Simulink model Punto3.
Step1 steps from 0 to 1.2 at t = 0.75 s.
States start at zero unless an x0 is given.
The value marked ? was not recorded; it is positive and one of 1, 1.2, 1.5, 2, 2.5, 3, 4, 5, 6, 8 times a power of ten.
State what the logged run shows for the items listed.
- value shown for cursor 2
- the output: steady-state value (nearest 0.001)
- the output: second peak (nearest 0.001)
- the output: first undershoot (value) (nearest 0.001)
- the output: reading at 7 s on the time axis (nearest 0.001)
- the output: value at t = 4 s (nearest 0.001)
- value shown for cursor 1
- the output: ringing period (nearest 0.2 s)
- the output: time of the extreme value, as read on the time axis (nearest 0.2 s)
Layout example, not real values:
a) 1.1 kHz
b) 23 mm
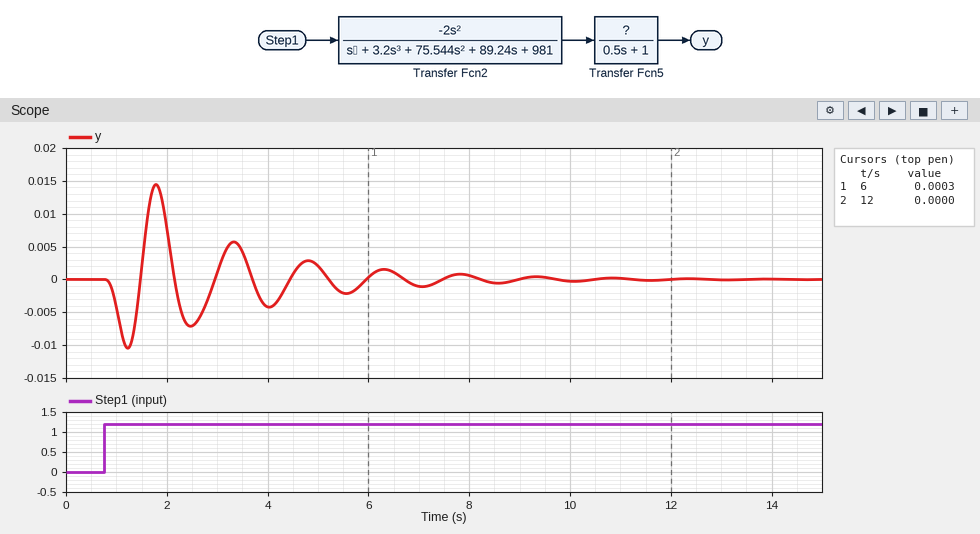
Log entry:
a) 0.0000
b) 0.000
c) 0.006
d) -0.007
e) -0.001
f) -0.004
g) 0.0003
h) 1.6 s
i) 1.8 s
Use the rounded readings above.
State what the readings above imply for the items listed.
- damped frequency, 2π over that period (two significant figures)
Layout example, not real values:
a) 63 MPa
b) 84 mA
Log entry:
a) 3.9 rad/s
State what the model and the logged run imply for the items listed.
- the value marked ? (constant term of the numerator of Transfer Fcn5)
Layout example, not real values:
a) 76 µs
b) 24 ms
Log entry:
a) 0.6
